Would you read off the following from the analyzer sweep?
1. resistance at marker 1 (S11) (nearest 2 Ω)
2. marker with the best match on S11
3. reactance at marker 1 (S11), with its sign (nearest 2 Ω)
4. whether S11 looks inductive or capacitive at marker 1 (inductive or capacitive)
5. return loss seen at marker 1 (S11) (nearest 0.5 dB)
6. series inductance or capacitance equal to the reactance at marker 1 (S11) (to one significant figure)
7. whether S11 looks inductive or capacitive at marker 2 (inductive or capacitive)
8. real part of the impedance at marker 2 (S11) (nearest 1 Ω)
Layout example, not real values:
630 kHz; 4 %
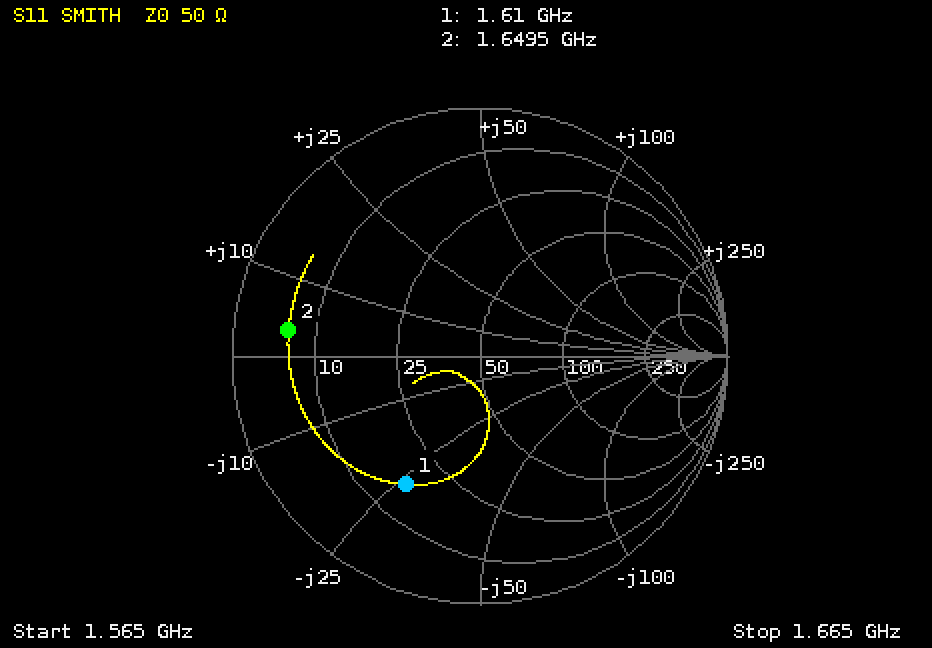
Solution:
16 Ω; marker 1; -26 Ω; capacitive; 4.5 dB; 4 pF; inductive; 6 Ω
